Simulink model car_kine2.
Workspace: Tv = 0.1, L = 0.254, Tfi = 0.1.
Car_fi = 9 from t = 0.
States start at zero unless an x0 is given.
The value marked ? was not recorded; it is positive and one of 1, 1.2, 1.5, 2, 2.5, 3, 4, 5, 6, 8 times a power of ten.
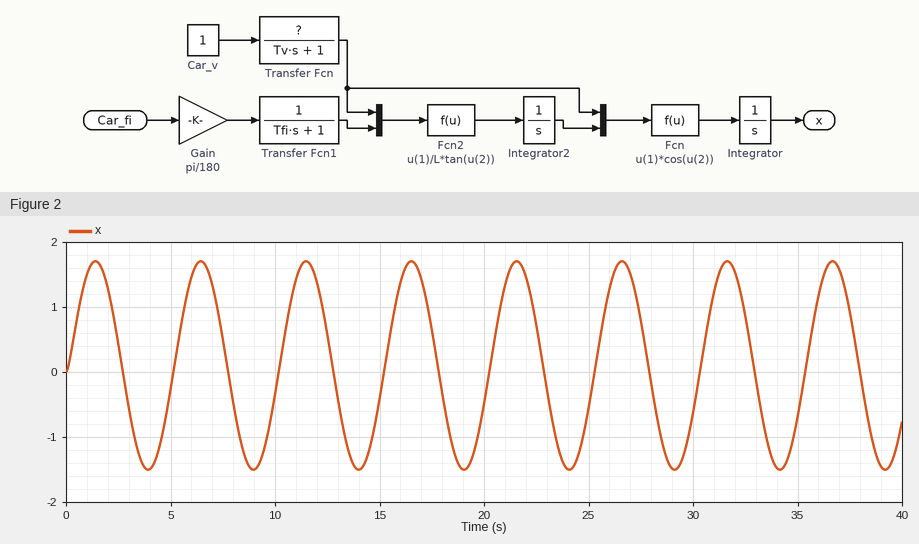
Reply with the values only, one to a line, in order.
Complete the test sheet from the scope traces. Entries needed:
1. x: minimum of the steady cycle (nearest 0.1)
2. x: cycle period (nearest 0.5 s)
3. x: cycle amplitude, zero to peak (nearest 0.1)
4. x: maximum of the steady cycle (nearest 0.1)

-1.5
5.0 s
1.6
1.7
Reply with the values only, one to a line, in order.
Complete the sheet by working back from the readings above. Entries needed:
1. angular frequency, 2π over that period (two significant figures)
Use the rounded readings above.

1.3 rad/s
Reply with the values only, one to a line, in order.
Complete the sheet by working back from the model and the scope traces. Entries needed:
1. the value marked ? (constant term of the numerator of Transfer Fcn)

2
